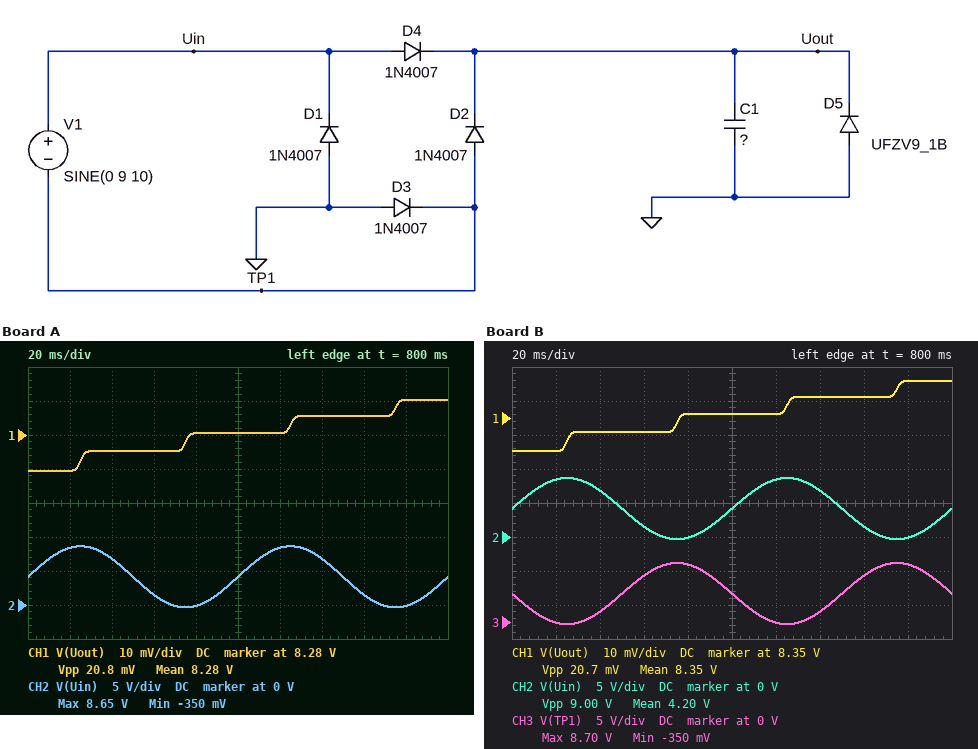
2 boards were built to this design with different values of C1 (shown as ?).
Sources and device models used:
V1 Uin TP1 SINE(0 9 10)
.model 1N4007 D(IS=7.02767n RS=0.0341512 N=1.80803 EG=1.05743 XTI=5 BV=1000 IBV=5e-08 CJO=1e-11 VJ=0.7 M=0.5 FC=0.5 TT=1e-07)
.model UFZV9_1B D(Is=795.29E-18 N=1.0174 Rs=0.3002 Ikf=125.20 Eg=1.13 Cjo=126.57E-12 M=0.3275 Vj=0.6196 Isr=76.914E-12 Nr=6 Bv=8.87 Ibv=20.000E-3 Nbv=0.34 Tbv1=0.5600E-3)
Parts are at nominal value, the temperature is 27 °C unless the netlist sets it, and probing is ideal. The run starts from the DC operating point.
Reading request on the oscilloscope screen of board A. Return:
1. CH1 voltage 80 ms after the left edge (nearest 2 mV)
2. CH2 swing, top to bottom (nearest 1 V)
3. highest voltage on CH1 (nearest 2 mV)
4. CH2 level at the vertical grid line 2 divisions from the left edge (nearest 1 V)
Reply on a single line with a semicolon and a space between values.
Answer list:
8.280 V; 9 V; 8.290 V; 7 V
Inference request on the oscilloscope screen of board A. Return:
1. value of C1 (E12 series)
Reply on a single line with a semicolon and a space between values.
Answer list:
12 µF
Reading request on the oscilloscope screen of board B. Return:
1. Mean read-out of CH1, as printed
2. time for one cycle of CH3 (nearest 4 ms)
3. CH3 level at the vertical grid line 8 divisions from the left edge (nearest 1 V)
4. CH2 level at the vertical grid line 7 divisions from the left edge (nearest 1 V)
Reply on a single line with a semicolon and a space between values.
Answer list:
8.35 V; 100 ms; 7 V; 7 V
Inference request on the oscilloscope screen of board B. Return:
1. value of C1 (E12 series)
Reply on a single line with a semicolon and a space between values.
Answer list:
5.6 µF
